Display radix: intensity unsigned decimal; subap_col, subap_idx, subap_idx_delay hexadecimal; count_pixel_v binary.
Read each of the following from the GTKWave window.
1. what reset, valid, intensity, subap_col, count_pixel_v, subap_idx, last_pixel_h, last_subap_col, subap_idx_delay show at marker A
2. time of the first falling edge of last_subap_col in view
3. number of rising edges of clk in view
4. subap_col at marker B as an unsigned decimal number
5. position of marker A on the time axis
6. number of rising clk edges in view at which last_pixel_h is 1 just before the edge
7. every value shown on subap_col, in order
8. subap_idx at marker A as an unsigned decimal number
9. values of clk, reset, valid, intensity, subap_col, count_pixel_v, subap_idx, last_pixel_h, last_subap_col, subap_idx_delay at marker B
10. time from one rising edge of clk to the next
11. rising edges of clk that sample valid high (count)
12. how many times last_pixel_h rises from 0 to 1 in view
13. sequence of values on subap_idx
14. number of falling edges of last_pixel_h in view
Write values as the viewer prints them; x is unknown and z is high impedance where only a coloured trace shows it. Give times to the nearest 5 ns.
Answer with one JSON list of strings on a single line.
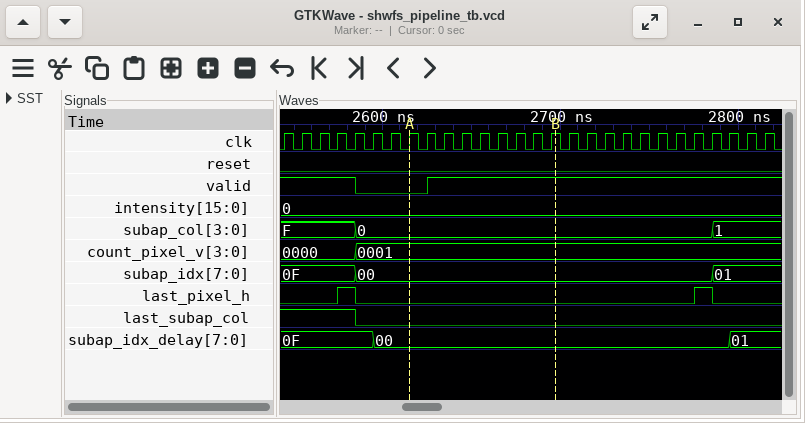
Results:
["reset=0, valid=0, intensity=0, subap_col=0, count_pixel_v=0001, subap_idx=00, last_pixel_h=0, last_subap_col=0, subap_idx_delay=00", "2585 ns", "28", "0", "2615 ns", "2", "F, 0, 1", "0", "clk=1, reset=0, valid=1, intensity=0, subap_col=0, count_pixel_v=0001, subap_idx=00, last_pixel_h=0, last_subap_col=0, subap_idx_delay=00", "10 ns", "24", "2", "0F, 00, 01", "2"]
